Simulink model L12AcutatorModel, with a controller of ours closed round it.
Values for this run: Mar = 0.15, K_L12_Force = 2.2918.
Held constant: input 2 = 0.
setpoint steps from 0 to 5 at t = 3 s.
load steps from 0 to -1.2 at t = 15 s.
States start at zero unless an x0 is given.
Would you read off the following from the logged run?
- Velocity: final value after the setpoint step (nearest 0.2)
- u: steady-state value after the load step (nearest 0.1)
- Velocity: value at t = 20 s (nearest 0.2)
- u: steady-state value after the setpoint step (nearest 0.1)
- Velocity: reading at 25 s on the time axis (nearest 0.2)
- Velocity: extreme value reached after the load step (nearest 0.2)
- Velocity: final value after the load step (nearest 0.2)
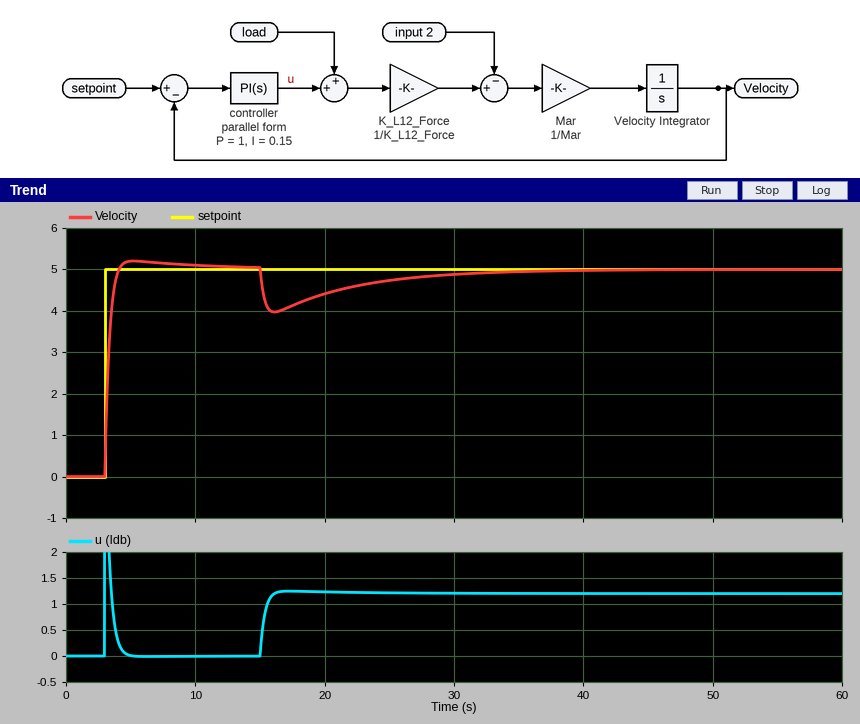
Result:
5.0
1.2
4.4
0.0
4.8
4.0
5.0
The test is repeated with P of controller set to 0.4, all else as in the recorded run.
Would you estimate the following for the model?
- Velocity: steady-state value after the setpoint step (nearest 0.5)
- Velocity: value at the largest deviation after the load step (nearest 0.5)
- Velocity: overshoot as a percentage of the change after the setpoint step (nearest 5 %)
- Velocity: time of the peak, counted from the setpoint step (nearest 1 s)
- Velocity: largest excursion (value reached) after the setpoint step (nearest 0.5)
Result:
5.0
3.0
15 %
3 s
6.0
